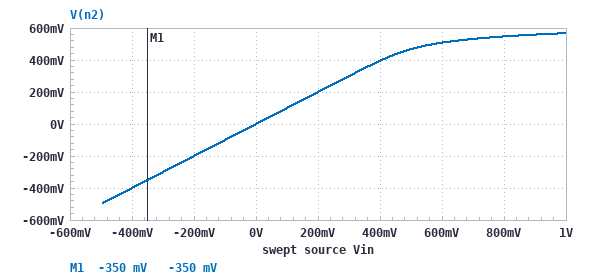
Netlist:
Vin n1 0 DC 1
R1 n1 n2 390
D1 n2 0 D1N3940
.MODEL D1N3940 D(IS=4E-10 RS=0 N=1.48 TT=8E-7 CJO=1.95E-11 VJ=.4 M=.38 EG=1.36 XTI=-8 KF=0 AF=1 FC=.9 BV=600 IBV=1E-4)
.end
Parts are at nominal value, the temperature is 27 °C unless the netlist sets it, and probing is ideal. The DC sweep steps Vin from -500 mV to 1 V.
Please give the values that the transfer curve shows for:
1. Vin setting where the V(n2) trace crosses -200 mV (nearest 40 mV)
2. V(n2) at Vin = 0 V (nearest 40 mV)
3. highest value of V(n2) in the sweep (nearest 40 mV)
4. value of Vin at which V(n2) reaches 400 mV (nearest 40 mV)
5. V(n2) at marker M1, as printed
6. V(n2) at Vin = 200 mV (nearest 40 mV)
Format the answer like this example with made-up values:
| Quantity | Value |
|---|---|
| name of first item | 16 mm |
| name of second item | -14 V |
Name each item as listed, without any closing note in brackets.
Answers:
| Quantity | Value |
|---|---|
| Vin setting where the V(n2) trace crosses -200 mV | -200 mV |
| V(n2) at Vin = 0 V | 0 V |
| highest value of V(n2) in the sweep | 560 mV |
| value of Vin at which V(n2) reaches 400 mV | 400 mV |
| V(n2) at marker M1, as printed | -350 mV |
| V(n2) at Vin = 200 mV | 200 mV |
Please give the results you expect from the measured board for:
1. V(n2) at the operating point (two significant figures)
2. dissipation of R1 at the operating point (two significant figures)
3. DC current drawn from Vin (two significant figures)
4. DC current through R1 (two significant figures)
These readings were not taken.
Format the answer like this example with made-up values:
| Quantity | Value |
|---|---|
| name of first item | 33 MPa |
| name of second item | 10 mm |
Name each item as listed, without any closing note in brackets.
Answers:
| Quantity | Value |
|---|---|
| V(n2) at the operating point | 570 mV |
| dissipation of R1 at the operating point | 480 µW |
| DC current drawn from Vin | 1.1 mA |
| DC current through R1 | 1.1 mA |
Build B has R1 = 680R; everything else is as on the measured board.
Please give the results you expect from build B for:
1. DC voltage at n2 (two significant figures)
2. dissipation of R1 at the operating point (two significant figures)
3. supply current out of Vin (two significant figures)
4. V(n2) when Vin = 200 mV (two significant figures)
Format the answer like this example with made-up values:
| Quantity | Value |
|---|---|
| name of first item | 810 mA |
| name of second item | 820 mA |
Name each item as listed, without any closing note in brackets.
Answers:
| Quantity | Value |
|---|---|
| DC voltage at n2 | 550 mV |
| dissipation of R1 at the operating point | 300 µW |
| supply current out of Vin | 660 µA |
| V(n2) when Vin = 200 mV | 200 mV |
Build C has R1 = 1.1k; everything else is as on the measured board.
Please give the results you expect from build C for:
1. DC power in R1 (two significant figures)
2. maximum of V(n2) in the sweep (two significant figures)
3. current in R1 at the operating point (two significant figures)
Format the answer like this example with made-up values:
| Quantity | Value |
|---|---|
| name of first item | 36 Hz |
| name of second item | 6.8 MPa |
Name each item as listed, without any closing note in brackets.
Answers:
| Quantity | Value |
|---|---|
| DC power in R1 | 200 µW |
| maximum of V(n2) in the sweep | 530 mV |
| current in R1 at the operating point | 430 µA |
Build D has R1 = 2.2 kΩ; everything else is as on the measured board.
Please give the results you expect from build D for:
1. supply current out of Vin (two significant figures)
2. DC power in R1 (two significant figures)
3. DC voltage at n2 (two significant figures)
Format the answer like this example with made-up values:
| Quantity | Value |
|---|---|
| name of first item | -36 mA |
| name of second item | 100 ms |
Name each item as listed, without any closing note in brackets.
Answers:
| Quantity | Value |
|---|---|
| supply current out of Vin | 220 µA |
| DC power in R1 | 110 µW |
| DC voltage at n2 | 510 mV |
